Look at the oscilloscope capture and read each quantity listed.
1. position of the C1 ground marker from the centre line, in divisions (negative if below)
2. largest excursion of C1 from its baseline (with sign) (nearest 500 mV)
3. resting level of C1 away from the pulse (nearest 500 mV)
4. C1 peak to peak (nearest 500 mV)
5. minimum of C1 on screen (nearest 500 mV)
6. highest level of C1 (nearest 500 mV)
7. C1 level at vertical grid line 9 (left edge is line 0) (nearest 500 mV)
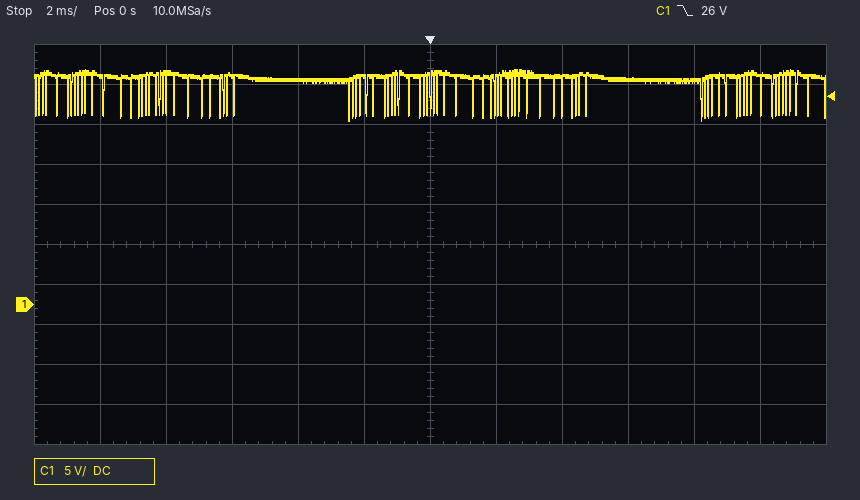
-1.5 div
-5.5 V
28.5 V
6.5 V
23.0 V
29.5 V
28.0 V
